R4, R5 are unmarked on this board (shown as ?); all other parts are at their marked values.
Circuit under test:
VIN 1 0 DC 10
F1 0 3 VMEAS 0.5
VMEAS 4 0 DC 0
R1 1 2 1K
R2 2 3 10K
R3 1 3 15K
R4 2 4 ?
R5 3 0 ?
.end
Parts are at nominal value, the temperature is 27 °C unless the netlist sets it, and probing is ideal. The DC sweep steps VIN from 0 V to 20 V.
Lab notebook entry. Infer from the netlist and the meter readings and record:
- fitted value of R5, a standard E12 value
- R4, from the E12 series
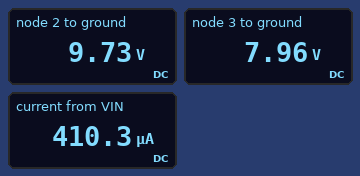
22 kΩ
100 kΩ
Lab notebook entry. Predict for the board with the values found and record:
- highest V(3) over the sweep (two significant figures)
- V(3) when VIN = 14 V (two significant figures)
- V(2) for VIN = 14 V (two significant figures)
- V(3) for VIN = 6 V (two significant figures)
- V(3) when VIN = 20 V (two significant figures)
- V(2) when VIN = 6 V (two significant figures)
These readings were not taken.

16 V
11 V
14 V
4.8 V
16 V
5.8 V
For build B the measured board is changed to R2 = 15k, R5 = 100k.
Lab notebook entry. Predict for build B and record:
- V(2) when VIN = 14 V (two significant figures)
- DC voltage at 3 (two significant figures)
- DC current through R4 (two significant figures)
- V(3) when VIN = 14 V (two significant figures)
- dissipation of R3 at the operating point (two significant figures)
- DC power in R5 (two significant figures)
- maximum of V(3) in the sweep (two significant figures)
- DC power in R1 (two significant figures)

14 V
9.6 V
99 µA
13 V
11 µW
920 µW
19 V
14 µW
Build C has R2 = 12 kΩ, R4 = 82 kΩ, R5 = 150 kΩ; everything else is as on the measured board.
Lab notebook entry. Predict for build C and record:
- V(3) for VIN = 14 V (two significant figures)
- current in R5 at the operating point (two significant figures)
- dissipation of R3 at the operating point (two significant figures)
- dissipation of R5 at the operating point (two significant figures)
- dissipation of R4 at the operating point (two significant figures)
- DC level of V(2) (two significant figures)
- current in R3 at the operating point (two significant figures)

14 V
66 µA
730 nW
650 µW
1.2 mW
9.9 V
7.0 µA
